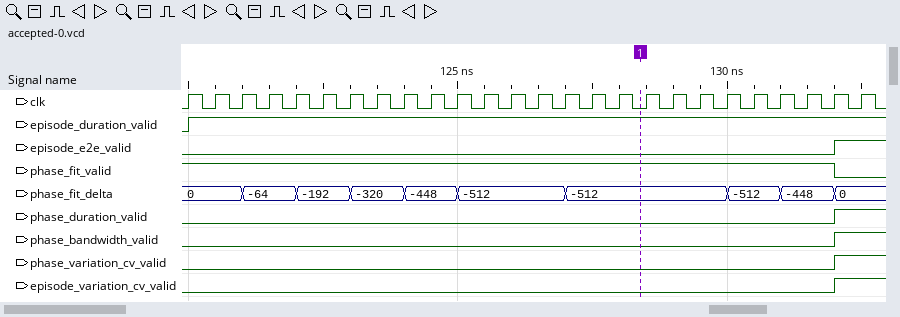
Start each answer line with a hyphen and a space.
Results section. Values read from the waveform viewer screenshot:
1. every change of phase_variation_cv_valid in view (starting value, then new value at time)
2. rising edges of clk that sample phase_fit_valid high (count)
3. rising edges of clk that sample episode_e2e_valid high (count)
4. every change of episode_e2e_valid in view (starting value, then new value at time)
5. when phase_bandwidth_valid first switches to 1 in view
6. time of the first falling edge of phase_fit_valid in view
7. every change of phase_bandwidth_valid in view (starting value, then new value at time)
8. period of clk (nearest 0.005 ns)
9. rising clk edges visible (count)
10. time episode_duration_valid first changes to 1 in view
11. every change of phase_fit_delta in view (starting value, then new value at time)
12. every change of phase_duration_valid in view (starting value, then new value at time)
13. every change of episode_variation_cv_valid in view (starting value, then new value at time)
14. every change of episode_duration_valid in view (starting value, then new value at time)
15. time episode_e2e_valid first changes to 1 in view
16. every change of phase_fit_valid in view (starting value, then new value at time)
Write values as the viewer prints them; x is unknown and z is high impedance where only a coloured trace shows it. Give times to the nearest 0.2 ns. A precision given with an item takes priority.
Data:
- 0, 1 at 132 ns
- 25
- 1
- 0, 1 at 132 ns
- 132 ns
- 132 ns
- 0, 1 at 132 ns
- 0.5 ns
- 26
- 120 ns
- 0, -64 at 121 ns, -192 at 122 ns, -320 at 123 ns, -448 at 124 ns, -512 at 125 ns, -512 at 127 ns, -512 at 130 ns, -448 at 131 ns, 0 at 132 ns
- 0, 1 at 132 ns
- 0, 1 at 132 ns
- 0, 1 at 120 ns
- 132 ns
- 1, 0 at 132 ns
